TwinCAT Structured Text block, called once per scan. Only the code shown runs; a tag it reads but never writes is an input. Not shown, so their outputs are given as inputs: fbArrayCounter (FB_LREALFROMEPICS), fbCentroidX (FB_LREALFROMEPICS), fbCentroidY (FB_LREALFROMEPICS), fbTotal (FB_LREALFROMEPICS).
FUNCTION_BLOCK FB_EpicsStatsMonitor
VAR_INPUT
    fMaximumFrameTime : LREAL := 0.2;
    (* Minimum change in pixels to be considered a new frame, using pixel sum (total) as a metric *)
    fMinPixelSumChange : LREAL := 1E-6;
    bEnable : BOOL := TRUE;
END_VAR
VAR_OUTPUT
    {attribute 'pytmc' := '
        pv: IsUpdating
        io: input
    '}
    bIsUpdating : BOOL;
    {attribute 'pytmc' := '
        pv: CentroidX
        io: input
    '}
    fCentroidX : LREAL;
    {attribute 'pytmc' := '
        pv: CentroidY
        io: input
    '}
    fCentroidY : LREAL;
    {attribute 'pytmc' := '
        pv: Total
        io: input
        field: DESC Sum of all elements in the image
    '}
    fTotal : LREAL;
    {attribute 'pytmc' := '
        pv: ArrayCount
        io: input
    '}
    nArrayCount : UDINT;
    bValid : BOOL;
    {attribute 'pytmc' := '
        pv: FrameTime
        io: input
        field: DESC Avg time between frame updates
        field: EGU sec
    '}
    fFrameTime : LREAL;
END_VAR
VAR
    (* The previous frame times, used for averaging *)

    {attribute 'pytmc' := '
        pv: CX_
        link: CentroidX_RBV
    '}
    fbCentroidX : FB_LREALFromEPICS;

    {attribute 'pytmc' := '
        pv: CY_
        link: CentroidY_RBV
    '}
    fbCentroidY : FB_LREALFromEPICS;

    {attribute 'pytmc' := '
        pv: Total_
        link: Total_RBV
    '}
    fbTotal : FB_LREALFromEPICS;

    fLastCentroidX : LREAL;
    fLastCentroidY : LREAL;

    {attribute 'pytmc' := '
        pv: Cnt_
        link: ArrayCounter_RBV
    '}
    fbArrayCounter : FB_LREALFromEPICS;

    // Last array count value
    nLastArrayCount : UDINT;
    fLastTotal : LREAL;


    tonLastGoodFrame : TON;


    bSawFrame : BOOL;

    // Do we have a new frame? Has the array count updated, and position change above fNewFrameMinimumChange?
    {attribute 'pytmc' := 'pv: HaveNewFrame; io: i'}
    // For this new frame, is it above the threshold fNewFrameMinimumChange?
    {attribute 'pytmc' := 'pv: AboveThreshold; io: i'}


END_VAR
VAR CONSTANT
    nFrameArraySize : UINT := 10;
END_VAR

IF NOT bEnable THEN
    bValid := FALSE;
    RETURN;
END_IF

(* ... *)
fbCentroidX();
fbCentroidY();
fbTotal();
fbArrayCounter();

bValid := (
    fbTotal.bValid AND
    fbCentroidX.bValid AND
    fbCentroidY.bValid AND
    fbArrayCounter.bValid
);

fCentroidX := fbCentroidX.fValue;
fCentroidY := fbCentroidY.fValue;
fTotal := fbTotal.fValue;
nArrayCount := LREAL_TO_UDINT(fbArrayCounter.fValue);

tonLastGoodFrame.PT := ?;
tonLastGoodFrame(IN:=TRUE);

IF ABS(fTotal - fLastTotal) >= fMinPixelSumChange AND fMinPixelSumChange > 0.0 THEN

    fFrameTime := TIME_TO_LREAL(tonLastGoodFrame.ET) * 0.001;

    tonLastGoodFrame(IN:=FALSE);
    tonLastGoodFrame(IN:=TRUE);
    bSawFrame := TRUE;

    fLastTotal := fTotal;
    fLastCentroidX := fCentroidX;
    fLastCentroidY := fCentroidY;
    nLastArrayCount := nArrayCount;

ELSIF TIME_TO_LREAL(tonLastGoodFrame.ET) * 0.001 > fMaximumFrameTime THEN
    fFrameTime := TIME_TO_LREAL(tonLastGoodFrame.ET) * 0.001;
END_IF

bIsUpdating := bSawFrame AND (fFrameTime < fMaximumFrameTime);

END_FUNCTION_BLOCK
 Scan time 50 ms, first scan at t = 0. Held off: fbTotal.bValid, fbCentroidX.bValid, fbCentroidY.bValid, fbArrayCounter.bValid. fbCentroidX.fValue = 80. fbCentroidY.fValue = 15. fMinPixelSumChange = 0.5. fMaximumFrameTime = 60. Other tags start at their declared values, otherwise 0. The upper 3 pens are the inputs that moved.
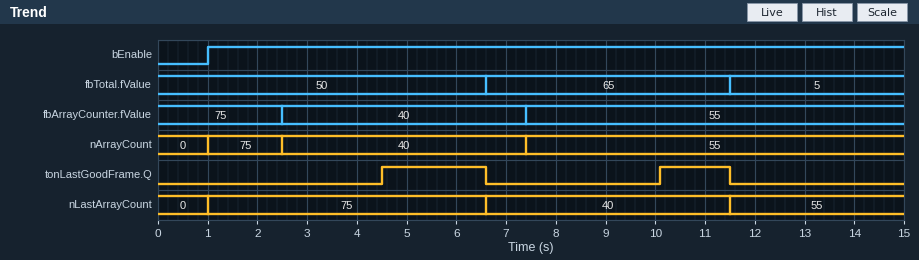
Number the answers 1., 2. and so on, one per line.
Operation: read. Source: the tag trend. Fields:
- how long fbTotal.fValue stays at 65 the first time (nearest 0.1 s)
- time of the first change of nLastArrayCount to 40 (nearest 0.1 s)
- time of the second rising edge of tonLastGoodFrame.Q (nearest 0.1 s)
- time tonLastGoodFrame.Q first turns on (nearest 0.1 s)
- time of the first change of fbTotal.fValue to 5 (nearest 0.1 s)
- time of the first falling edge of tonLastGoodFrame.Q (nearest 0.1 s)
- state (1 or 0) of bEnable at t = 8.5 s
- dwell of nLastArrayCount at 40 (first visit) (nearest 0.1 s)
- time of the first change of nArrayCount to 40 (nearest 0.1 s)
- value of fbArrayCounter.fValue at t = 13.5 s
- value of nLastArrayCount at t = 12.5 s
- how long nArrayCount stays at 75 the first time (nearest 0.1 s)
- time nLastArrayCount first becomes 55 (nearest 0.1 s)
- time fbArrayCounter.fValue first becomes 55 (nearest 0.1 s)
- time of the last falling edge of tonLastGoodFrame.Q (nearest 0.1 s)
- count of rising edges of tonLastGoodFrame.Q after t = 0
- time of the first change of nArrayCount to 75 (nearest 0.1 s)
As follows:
1. 4.9 s
2. 6.6 s
3. 10.1 s
4. 4.5 s
5. 11.5 s
6. 6.6 s
7. 1
8. 4.9 s
9. 2.5 s
10. 55
11. 55
12. 1.5 s
13. 11.5 s
14. 7.4 s
15. 11.5 s
16. 2
17. 1.0 s
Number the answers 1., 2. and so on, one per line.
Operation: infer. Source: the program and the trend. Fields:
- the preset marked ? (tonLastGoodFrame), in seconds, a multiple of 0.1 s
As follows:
1. 3.5 s
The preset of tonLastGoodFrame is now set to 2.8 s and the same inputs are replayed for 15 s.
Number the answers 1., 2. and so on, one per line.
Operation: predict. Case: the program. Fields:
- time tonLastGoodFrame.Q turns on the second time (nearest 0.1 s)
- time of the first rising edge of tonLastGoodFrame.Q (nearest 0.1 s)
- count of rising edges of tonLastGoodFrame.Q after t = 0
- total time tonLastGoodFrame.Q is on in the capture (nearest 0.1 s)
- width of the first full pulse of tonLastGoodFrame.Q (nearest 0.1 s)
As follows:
1. 9.4 s
2. 3.8 s
3. 3
4. 5.6 s
5. 2.8 s
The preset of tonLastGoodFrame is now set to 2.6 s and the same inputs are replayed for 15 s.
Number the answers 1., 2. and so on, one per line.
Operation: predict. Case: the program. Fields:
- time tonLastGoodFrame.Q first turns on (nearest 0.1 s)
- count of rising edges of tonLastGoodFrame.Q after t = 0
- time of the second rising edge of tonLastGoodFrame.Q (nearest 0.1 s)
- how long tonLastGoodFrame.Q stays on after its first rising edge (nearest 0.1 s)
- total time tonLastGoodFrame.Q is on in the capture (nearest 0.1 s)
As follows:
1. 3.6 s
2. 3
3. 9.2 s
4. 3.0 s
5. 6.2 s
